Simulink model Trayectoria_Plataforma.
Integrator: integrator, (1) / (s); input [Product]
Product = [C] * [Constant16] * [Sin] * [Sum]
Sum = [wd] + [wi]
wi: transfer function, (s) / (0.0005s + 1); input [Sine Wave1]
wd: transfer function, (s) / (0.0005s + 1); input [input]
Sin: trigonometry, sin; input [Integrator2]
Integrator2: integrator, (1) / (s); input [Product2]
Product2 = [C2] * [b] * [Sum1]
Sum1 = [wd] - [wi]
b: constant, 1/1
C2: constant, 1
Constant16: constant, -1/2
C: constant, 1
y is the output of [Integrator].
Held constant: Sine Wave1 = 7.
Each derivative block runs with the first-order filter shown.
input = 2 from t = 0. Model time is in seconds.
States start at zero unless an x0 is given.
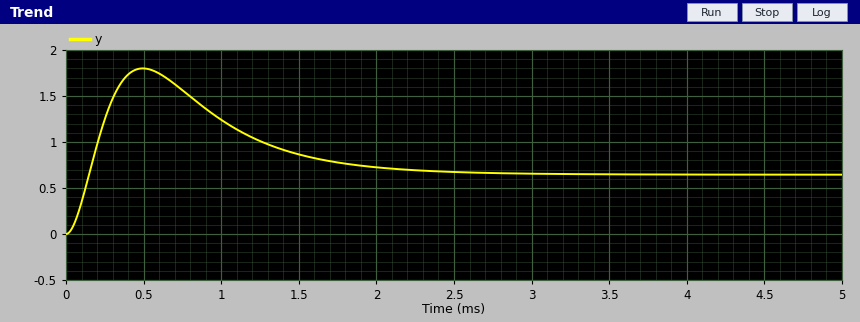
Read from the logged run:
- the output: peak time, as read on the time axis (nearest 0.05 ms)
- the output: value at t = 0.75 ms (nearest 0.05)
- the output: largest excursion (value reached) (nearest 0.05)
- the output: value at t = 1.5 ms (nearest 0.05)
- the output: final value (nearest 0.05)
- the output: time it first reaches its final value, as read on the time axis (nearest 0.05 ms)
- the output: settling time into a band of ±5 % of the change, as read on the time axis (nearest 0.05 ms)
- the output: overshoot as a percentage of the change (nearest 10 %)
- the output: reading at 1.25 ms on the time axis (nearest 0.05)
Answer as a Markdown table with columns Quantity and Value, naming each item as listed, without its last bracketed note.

| Quantity | Value |
|---|---|
| the output: peak time, as read on the time axis | 0.50 ms |
| the output: value at t = 0.75 ms | 1.55 |
| the output: largest excursion (value reached) | 1.80 |
| the output: value at t = 1.5 ms | 0.85 |
| the output: final value | 0.65 |
| the output: time it first reaches its final value, as read on the time axis | 0.15 ms |
| the output: settling time into a band of ±5 % of the change, as read on the time axis | 2.45 ms |
| the output: overshoot as a percentage of the change | 180 % |
| the output: reading at 1.25 ms on the time axis | 1.00 |
